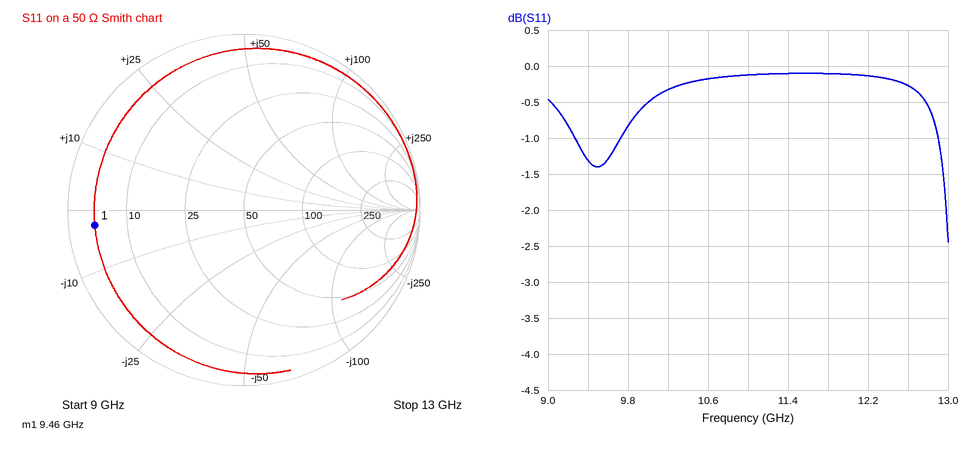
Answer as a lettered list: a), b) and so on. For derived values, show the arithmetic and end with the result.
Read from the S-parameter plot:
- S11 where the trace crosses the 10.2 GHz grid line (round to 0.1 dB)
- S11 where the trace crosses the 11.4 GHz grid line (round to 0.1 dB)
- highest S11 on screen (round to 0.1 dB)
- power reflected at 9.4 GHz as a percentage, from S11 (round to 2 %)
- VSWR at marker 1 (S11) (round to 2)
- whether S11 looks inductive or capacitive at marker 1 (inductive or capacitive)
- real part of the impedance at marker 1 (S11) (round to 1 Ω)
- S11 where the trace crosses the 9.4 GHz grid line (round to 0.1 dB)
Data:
a) -0.3 dB
b) -0.1 dB
c) -0.1 dB
d) 10^(-1.3/10) ≈ 74 %
e) 12
f) capacitive
g) 4 Ω
h) -1.3 dB
